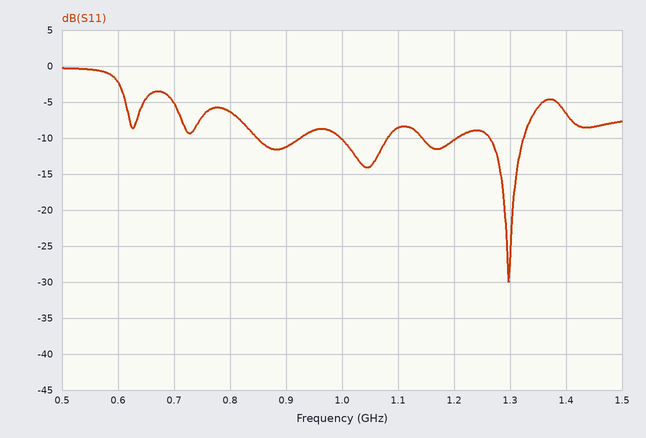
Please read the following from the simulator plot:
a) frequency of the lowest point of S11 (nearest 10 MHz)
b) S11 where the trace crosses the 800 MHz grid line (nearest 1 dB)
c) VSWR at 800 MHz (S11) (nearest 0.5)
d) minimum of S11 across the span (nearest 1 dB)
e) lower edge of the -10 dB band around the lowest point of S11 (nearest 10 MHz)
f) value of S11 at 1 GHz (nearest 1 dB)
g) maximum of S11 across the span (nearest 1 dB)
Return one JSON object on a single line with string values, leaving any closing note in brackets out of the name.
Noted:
{"frequency of the lowest point of S11": "1.30 GHz", "S11 where the trace crosses the 800 MHz grid line": "-6 dB", "VSWR at 800 MHz (S11)": "3.0", "minimum of S11 across the span": "-30 dB", "lower edge of the -10 dB band around the lowest point of S11": "1.26 GHz", "value of S11 at 1 GHz": "-10 dB", "maximum of S11 across the span": "0 dB"}
